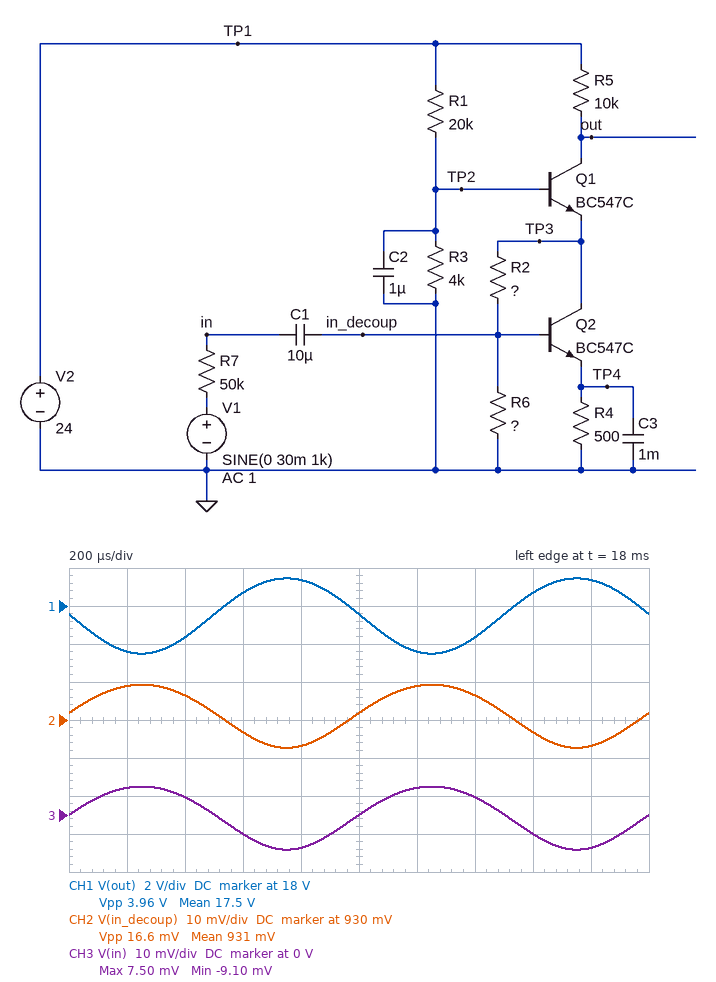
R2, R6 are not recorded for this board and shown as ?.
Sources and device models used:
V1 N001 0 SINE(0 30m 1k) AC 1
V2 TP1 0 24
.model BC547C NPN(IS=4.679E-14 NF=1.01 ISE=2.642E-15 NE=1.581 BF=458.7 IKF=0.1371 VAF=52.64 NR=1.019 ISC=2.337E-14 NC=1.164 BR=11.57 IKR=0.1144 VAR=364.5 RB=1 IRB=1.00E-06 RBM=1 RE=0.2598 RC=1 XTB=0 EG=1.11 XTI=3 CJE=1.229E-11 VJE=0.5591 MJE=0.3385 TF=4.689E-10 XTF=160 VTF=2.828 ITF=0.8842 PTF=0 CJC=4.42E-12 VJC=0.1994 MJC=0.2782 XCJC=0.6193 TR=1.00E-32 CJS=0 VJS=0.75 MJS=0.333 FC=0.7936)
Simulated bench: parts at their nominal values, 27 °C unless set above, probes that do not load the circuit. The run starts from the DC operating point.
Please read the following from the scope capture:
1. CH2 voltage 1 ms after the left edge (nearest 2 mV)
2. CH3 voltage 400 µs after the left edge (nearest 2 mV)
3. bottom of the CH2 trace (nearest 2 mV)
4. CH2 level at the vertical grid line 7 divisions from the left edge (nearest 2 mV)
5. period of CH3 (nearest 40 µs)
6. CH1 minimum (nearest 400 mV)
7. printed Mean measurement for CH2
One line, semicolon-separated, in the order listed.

932 mV; 4 mV; 922 mV; 936 mV; 1.00 ms; 15.6 V; 931 mV
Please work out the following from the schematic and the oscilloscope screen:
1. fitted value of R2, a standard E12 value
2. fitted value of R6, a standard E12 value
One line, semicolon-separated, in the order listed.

1.5 MΩ; 3.3 MΩ
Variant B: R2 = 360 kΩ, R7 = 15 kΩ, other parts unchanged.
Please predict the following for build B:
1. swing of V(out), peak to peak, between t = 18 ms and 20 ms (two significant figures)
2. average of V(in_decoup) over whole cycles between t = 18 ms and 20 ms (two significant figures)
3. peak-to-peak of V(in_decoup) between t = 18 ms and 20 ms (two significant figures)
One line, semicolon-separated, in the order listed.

8.5 V; 1.6 V; 18 mV
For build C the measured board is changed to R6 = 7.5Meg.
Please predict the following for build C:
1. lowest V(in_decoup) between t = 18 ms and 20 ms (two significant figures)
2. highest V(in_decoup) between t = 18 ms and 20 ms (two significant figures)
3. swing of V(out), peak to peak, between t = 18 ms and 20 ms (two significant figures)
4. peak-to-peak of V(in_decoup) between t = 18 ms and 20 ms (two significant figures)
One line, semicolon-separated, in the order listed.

960 mV; 970 mV; 4.1 V; 16 mV
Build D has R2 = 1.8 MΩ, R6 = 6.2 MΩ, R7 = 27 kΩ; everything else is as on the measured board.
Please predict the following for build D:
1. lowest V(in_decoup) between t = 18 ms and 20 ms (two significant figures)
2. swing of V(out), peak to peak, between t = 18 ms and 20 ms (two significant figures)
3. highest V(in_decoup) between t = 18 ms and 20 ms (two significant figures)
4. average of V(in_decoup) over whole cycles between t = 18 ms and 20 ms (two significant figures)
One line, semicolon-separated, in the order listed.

890 mV; 5.7 V; 910 mV; 900 mV
